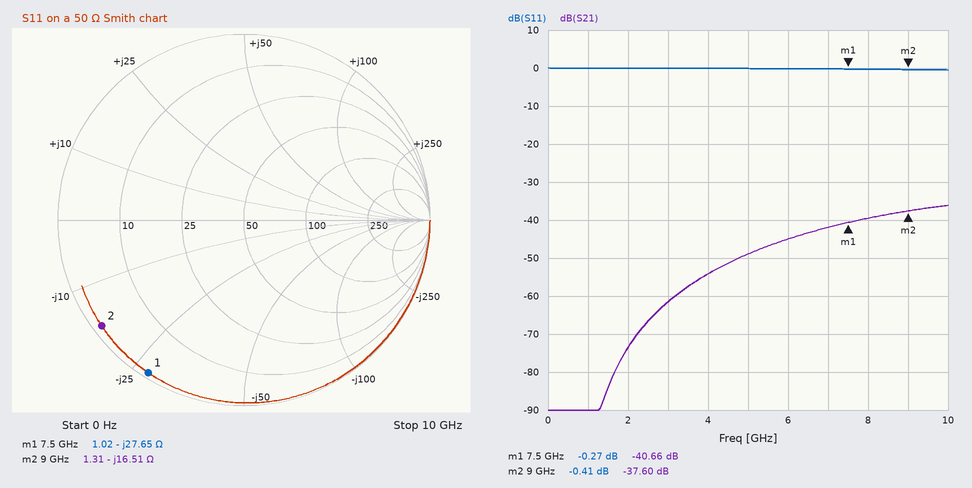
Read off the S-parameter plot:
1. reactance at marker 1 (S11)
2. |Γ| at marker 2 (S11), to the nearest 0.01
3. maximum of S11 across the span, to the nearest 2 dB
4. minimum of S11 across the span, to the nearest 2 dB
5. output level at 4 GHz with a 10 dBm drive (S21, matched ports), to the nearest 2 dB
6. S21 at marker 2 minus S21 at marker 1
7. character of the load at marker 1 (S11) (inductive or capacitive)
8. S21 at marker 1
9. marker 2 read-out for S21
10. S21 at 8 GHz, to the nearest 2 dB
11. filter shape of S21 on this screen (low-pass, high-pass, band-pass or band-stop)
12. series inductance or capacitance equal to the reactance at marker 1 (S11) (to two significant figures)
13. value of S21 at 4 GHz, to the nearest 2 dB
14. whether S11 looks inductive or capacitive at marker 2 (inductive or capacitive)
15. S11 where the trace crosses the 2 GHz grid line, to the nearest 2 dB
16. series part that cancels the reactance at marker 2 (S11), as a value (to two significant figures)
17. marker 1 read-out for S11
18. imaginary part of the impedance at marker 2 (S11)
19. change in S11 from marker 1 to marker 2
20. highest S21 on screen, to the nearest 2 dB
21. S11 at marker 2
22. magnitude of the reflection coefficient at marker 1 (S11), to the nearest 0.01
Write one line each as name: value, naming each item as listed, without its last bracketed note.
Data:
reactance at marker 1: -27.65 Ω
|Γ| at marker 2 (S11), to the nearest 0.01: 0.95
maximum of S11 across the span, to the nearest 2 dB: 0 dB
minimum of S11 across the span, to the nearest 2 dB: 0 dB
output level at 4 GHz with a 10 dBm drive (S21, matched ports), to the nearest 2 dB: -44 dBm
S21 at marker 2 minus S21 at marker 1: 3.06 dB
character of the load at marker 1 (S11): capacitive
S21 at marker 1: -40.66 dB
marker 2 read-out for S21: -37.60 dB
S21 at 8 GHz, to the nearest 2 dB: -40 dB
filter shape of S21 on this screen: high-pass
series inductance or capacitance equal to the reactance at marker 1 (S11): 770 fF
value of S21 at 4 GHz, to the nearest 2 dB: -54 dB
whether S11 looks inductive or capacitive at marker 2: capacitive
S11 where the trace crosses the 2 GHz grid line, to the nearest 2 dB: 0 dB
series part that cancels the reactance at marker 2 (S11), as a value: 290 pH
marker 1 read-out for S11: -0.27 dB
imaginary part of the impedance at marker 2: -16.51 Ω
change in S11 from marker 1 to marker 2: -0.14 dB
highest S21 on screen, to the nearest 2 dB: -36 dB
S11 at marker 2: -0.41 dB
magnitude of the reflection coefficient at marker 1 (S11), to the nearest 0.01: 0.97
